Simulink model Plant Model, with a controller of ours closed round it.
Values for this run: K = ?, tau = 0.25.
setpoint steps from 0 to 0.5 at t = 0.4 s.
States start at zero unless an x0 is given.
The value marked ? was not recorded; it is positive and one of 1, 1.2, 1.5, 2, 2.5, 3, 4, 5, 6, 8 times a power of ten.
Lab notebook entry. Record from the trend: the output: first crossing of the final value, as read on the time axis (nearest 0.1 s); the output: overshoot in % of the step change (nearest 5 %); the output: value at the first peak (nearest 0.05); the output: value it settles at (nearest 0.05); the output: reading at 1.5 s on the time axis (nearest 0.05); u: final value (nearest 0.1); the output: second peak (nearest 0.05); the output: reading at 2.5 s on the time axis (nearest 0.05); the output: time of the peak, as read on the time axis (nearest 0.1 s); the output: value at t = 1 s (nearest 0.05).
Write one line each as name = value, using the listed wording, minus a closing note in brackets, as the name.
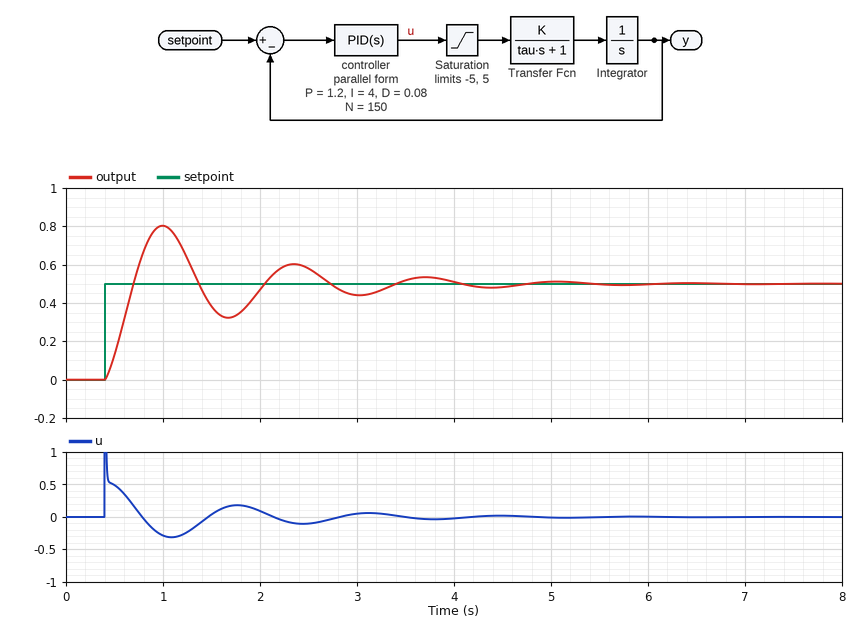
the output: first crossing of the final value, as read on the time axis = 0.7 s
the output: overshoot in % of the step change = 60 %
the output: value at the first peak = 0.80
the output: value it settles at = 0.50
the output: reading at 1.5 s on the time axis = 0.40
u: final value = 0.0
the output: second peak = 0.60
the output: reading at 2.5 s on the time axis = 0.60
the output: time of the peak, as read on the time axis = 1.0 s
the output: value at t = 1 s = 0.80
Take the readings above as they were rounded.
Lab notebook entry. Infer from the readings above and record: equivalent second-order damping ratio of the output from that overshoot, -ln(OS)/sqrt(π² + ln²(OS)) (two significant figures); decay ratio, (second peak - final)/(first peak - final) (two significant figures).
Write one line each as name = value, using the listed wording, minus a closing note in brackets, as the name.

equivalent second-order damping ratio of the output from that overshoot, -ln(OS)/sqrt(π² + ln²(OS)) = 0.16
decay ratio, (second peak - final)/(first peak - final) = 0.33
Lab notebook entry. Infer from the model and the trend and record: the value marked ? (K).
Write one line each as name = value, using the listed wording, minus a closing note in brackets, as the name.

the value marked ? = 6
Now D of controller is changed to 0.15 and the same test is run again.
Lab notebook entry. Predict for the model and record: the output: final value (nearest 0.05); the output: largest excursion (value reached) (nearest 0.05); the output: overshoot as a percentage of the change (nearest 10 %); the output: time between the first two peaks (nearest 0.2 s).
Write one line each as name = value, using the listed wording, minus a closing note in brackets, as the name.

the output: final value = 0.50
the output: largest excursion (value reached) = 0.75
the output: overshoot as a percentage of the change = 50 %
the output: time between the first two peaks = 1.6 s
